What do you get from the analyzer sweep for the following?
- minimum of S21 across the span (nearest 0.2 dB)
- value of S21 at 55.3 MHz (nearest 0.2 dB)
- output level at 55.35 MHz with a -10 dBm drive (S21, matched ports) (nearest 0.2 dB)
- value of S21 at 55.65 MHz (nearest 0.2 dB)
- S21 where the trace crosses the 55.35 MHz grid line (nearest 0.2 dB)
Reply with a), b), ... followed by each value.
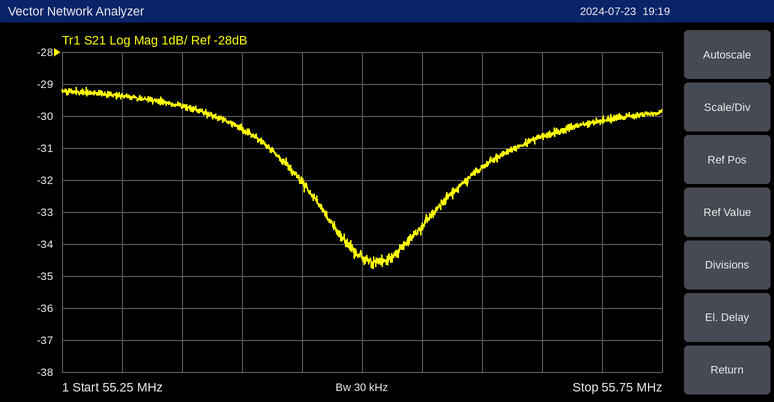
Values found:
a) -34.8 dB
b) -29.4 dB
c) -39.8 dBm
d) -30.6 dB
e) -29.8 dB
